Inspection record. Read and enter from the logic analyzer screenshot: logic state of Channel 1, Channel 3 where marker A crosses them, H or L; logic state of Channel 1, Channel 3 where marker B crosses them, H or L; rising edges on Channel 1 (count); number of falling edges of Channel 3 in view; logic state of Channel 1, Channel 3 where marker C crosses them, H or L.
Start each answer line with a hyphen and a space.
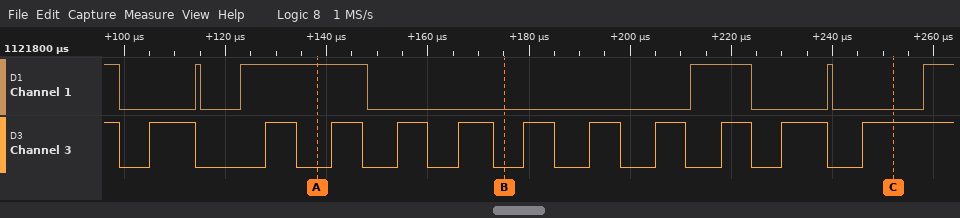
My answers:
- Channel 1=H, Channel 3=L
- Channel 1=L, Channel 3=L
- 5
- 11
- Channel 1=L, Channel 3=H
